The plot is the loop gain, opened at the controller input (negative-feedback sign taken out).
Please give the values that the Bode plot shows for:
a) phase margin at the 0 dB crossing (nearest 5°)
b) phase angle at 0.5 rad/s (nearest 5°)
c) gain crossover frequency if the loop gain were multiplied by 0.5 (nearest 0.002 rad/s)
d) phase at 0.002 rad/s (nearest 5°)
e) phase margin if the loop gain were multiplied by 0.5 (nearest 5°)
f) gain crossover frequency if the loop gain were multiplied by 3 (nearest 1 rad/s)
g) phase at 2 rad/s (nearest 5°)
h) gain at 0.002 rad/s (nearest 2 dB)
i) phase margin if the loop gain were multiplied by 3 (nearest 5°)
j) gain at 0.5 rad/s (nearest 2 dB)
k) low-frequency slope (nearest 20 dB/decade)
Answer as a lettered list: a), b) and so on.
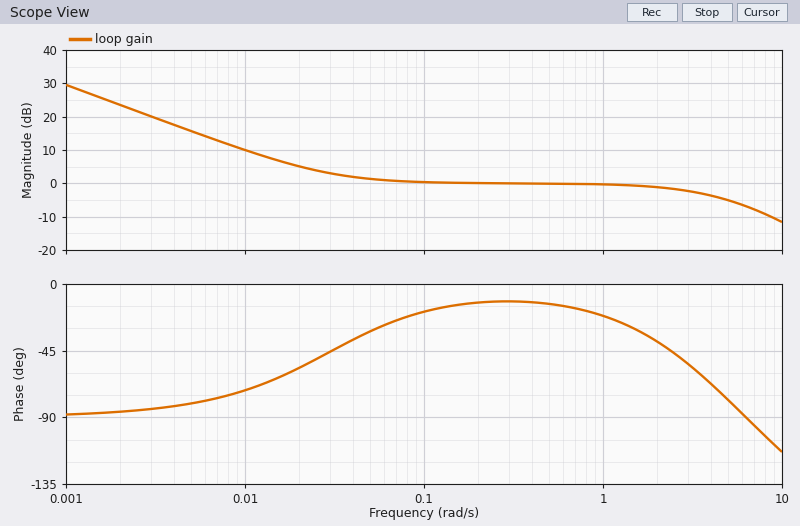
a) 170°
b) -15°
c) 0.018 rad/s
d) -85°
e) 120°
f) 8 rad/s
g) -40°
h) 24 dB
i) 75°
j) 0 dB
k) -20 dB/decade
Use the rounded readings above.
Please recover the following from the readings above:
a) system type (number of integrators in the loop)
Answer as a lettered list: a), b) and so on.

a) 1
